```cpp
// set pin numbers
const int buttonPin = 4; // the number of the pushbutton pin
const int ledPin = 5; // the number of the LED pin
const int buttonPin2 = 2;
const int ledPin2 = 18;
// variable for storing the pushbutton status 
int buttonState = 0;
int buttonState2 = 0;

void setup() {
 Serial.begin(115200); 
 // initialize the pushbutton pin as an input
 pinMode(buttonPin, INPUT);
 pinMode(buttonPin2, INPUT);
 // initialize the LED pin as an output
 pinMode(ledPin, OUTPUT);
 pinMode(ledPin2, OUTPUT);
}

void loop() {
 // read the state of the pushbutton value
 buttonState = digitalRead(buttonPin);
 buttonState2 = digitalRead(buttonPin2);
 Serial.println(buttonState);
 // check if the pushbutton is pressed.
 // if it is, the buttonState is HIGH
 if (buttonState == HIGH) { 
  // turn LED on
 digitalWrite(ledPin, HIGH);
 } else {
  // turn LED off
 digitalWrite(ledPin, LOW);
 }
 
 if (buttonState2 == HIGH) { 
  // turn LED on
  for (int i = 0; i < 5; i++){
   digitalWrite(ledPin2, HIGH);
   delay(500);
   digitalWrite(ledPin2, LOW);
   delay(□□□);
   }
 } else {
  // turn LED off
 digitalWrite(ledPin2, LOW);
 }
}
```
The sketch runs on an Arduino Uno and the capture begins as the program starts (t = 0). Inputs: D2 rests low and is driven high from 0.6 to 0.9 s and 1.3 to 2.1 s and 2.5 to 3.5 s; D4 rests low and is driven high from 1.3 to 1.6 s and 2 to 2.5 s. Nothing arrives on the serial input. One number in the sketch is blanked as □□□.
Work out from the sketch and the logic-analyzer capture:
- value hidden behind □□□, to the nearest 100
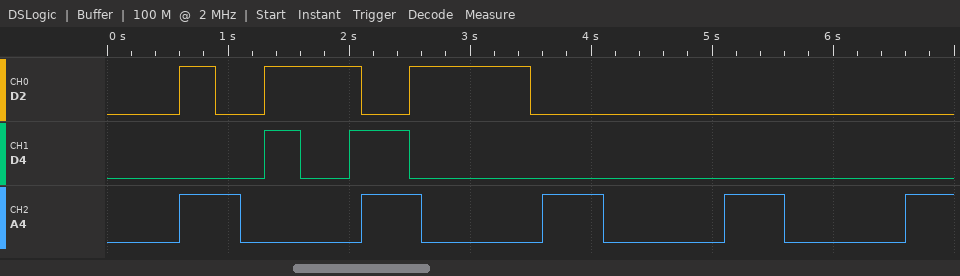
1000
